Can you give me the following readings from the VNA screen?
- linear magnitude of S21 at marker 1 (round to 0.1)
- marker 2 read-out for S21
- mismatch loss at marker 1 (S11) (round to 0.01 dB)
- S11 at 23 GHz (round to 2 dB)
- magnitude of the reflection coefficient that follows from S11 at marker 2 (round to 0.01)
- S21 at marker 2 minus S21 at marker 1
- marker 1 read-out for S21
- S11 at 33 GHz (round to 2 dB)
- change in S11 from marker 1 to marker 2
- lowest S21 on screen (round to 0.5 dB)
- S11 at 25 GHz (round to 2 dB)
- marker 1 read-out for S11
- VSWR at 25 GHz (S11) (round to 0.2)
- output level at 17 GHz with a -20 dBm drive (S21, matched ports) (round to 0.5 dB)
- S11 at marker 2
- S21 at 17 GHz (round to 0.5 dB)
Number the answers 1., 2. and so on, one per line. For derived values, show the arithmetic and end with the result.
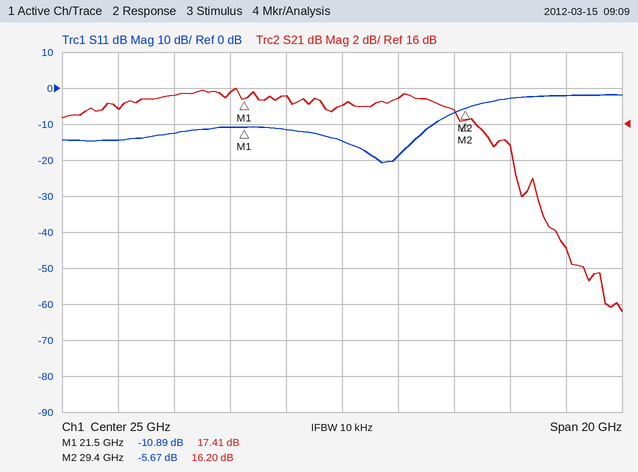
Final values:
1. 10^(17.41/20) ≈ 7.4
2. 16.20 dB
3. −10 log10(1 − 10^(-10.89/10)) ≈ 0.37 dB
4. -12 dB
5. 10^(-5.67/20) ≈ 0.52
6. 16.2 − (17.41) = -1.21 dB
7. 17.41 dB
8. -2 dB
9. -5.67 − (-10.89) = 5.22 dB
10. 5.5 dB
11. -14 dB
12. -10.89 dB
13. |Γ| = 10^(-14/20) = 0.1995; VSWR = (1 + 0.1995)/(1 − 0.1995) ≈ 1.50, so 1.4 to the nearest 0.2
14. -20 dBm + (17.0 dB) = -3.0 dBm
15. -5.67 dB
16. 17.0 dB
